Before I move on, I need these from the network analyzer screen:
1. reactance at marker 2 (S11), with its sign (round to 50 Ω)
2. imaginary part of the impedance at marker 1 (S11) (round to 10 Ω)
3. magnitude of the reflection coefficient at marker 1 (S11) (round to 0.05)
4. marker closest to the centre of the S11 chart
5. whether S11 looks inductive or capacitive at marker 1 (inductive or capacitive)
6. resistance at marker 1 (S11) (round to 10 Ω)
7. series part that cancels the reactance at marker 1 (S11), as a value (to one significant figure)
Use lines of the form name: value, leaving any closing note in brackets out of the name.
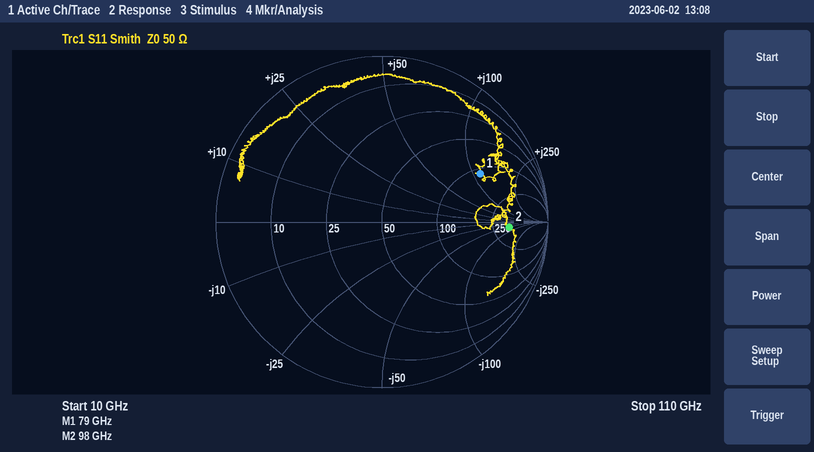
reactance at marker 2 (S11), with its sign: -50 Ω
imaginary part of the impedance at marker 1 (S11): +120 Ω
magnitude of the reflection coefficient at marker 1 (S11): 0.65
marker closest to the centre of the S11 chart: marker 1
whether S11 looks inductive or capacitive at marker 1: inductive
resistance at marker 1 (S11): 110 Ω
series part that cancels the reactance at marker 1 (S11), as a value: 20 fF
